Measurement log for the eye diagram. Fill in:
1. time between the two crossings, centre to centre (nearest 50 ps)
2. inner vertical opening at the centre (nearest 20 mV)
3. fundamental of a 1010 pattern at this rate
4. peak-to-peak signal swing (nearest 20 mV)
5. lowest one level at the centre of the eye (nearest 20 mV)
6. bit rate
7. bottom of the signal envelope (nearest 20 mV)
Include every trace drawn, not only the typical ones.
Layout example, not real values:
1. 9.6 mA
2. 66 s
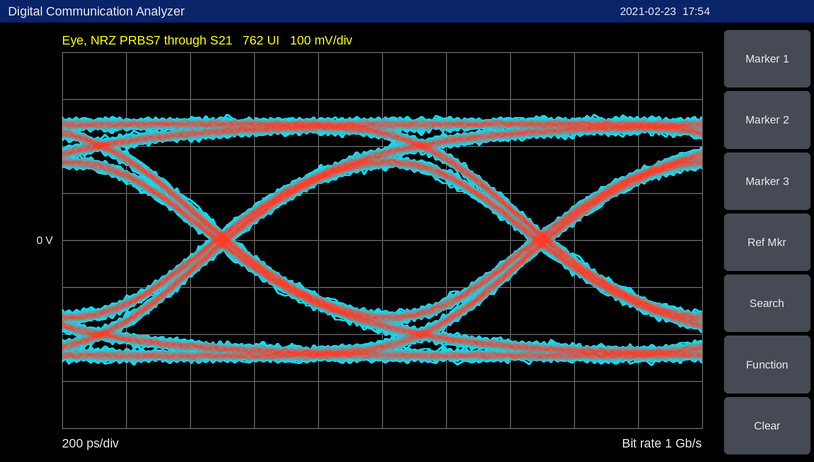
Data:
1. 1.00 ns
2. 300 mV
3. 500 MHz
4. 540 mV
5. 160 mV
6. 1 Gb/s
7. -260 mV
